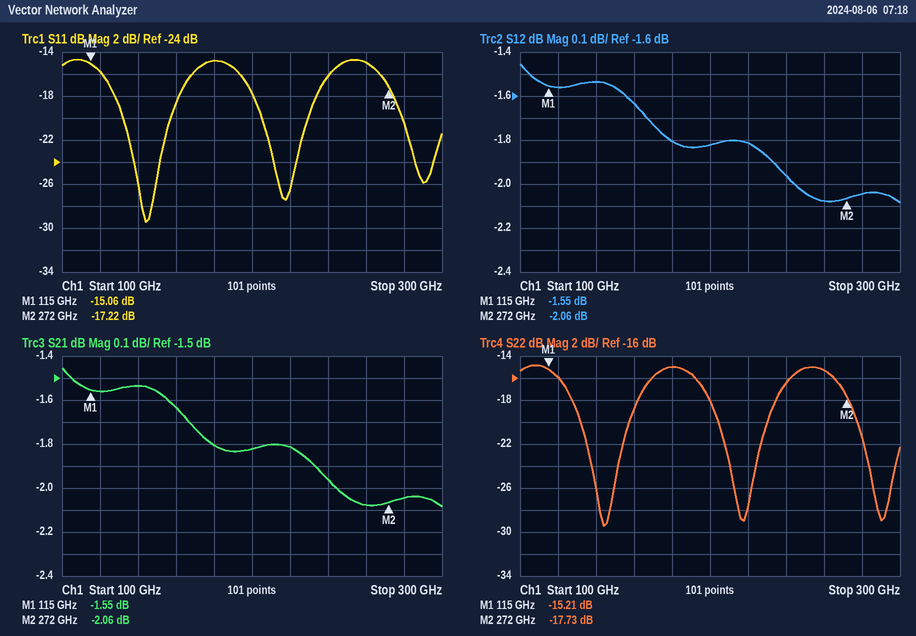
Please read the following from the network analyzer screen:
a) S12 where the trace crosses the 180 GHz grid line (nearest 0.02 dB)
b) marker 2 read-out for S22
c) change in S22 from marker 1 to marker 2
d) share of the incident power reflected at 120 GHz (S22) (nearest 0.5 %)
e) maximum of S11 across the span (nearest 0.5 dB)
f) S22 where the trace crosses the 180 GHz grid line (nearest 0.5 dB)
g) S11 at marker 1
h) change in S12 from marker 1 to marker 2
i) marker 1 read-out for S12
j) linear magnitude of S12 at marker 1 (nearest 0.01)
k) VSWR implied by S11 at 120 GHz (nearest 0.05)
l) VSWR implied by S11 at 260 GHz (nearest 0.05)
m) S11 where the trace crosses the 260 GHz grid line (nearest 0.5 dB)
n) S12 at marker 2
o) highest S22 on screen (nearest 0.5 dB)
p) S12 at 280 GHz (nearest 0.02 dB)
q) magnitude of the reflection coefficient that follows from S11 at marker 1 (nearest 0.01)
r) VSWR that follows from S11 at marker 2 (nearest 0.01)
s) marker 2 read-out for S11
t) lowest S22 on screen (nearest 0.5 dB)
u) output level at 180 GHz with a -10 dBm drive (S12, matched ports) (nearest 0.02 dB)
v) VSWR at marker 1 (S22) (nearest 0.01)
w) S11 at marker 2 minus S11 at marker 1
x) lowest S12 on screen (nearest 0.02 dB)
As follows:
-1.80 dB
-17.73 dB
-2.52 dB
2.5 %
-14.5 dB
-15.0 dB
-15.06 dB
-0.51 dB
-1.55 dB
0.84
1.40
1.45
-15.0 dB
-2.06 dB
-15.0 dB
-2.04 dB
0.18
1.32
-17.22 dB
-29.5 dB
-11.80 dBm
1.42
-2.16 dB
-2.08 dB
